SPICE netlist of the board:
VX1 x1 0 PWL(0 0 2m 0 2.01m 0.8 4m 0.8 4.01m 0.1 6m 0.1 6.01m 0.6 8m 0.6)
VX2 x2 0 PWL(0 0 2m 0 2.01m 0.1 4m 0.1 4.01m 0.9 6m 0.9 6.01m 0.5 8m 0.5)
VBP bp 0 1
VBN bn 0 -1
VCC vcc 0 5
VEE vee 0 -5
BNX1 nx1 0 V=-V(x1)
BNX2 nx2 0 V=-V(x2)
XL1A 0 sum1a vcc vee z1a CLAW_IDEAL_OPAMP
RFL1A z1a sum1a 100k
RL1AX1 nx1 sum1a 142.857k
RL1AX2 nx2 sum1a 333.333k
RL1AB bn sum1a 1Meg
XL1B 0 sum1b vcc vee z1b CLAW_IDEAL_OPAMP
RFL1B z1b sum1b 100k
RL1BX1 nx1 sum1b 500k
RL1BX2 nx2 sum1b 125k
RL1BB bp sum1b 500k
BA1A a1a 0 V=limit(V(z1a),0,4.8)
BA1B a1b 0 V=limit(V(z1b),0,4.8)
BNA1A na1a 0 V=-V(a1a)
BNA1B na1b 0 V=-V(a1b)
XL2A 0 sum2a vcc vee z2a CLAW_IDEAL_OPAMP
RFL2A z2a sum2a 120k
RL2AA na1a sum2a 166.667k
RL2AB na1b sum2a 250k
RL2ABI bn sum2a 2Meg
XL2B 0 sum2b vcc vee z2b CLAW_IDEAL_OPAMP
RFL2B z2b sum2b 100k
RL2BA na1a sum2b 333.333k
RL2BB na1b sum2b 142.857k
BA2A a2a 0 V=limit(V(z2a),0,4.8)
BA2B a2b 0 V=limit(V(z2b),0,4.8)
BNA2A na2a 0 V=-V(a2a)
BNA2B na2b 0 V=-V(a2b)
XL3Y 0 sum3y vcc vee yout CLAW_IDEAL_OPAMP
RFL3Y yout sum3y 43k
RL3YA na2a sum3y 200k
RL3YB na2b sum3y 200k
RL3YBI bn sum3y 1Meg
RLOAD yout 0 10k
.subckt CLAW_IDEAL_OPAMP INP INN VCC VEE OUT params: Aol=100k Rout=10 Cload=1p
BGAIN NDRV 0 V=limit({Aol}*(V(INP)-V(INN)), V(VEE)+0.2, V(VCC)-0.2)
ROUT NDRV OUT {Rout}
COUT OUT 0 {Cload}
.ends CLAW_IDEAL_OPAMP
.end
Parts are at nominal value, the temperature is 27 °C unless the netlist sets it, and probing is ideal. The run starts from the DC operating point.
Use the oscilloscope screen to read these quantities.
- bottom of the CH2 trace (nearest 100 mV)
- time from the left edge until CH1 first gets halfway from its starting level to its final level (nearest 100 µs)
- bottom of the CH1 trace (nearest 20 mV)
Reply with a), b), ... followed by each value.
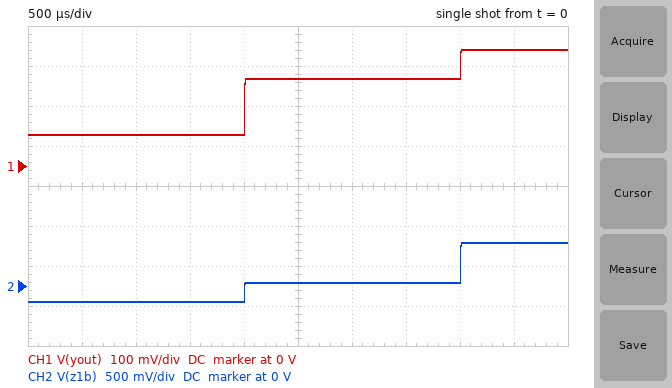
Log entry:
a) -200 mV
b) 2.0 ms
c) 80 mV
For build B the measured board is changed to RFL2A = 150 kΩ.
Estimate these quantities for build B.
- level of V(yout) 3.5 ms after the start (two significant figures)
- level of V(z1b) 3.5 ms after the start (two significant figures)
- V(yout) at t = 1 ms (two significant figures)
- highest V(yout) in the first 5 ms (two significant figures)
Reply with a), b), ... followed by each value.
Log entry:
a) 250 mV
b) 40 mV
c) 85 mV
d) 320 mV
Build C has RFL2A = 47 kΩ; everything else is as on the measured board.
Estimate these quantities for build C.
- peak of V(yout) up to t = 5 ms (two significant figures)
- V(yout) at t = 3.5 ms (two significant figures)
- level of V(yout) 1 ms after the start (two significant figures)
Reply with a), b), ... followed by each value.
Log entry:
a) 210 mV
b) 140 mV
c) 61 mV
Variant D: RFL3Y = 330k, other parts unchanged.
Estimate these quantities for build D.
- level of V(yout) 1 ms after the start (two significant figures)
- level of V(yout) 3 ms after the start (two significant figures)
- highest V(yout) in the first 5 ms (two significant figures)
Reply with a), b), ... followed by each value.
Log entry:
a) 600 mV
b) 1.7 V
c) 2.2 V
